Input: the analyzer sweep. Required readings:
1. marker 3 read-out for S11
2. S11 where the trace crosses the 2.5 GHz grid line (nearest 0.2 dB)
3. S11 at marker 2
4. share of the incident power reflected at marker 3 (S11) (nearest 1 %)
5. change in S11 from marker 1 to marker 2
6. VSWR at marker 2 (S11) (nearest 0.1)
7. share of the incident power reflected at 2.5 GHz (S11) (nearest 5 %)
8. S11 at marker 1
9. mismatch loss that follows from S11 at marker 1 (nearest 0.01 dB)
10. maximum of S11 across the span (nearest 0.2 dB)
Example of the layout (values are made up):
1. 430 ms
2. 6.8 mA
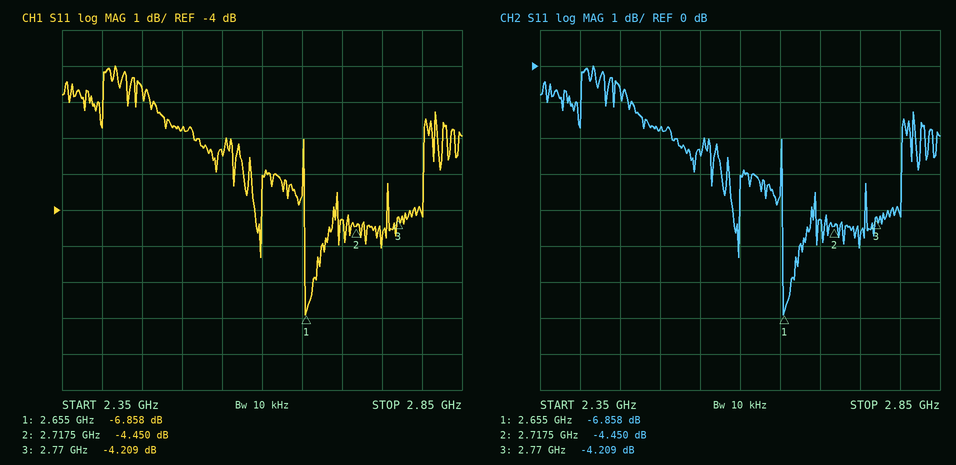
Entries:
1. -4.209 dB
2. -1.8 dB
3. -4.450 dB
4. 38 %
5. 2.408 dB
6. 4.0
7. 65 %
8. -6.858 dB
9. 1.00 dB
10. 0.0 dB
